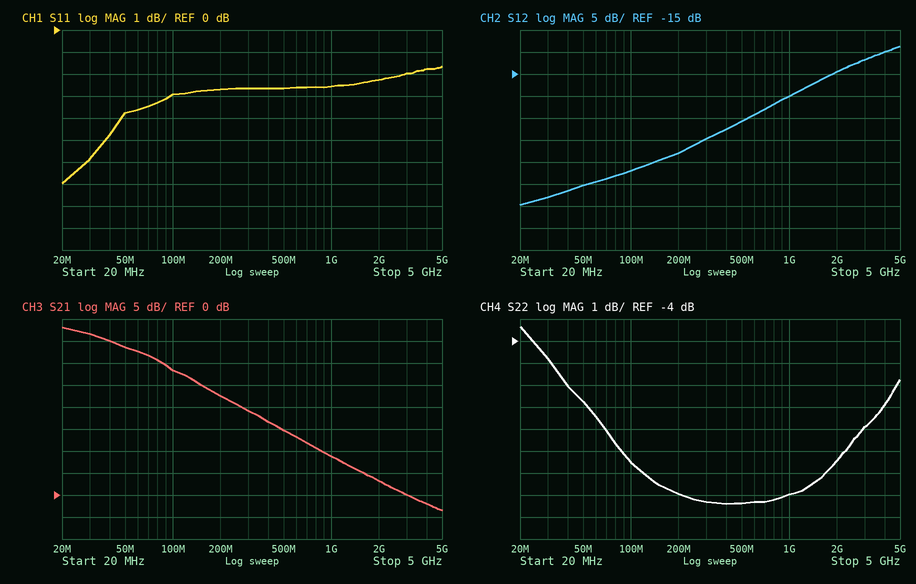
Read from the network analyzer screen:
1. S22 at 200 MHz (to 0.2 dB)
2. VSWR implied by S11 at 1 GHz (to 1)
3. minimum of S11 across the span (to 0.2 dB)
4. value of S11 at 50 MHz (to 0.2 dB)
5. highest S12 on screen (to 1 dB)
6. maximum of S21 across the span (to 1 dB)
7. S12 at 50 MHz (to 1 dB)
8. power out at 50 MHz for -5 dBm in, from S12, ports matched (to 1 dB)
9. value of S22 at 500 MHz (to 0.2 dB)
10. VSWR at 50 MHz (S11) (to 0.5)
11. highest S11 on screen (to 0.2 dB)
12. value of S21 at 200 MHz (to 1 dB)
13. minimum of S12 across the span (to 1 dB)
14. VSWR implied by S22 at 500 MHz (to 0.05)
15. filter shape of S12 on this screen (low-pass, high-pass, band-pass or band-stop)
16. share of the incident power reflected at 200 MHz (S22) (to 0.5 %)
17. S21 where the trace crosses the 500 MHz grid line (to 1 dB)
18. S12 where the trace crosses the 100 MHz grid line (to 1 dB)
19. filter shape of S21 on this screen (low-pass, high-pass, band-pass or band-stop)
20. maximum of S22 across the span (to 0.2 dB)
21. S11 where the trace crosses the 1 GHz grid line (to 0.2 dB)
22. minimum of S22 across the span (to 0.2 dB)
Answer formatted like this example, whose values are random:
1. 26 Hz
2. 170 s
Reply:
1. -11.0 dB
2. 7
3. -7.0 dB
4. -3.8 dB
5. -9 dB
6. 38 dB
7. -40 dB
8. -45 dBm
9. -11.4 dB
10. 4.5
11. -1.6 dB
12. 23 dB
13. -45 dB
14. 1.75
15. high-pass
16. 8.0 %
17. 15 dB
18. -37 dB
19. low-pass
20. -3.4 dB
21. -2.6 dB
22. -11.4 dB
